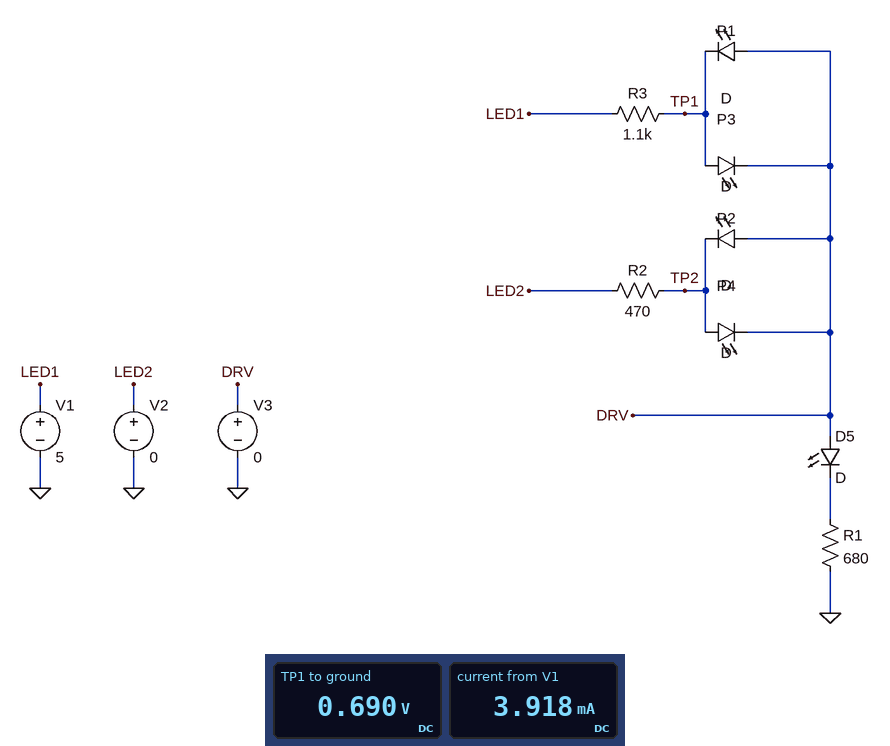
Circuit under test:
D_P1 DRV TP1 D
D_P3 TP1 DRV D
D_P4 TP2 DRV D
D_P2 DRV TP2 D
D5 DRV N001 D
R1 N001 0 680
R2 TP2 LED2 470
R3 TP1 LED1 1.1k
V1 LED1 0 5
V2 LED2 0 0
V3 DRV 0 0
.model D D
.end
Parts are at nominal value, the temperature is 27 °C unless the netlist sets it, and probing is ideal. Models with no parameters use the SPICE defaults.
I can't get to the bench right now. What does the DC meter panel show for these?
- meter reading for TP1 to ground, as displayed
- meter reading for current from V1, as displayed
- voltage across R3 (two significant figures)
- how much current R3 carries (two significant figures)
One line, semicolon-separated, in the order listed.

0.690 V; 3.918 mA; 4.3 V; 3.9 mA
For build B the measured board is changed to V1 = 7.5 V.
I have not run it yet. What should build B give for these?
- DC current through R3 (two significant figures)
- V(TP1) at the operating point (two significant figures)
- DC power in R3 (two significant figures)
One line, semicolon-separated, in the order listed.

6.2 mA; 700 mV; 42 mW
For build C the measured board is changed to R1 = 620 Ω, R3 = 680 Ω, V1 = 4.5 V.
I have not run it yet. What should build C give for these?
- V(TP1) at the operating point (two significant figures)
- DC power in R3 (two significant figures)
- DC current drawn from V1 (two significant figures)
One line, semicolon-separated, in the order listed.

700 mV; 21 mW; 5.6 mA
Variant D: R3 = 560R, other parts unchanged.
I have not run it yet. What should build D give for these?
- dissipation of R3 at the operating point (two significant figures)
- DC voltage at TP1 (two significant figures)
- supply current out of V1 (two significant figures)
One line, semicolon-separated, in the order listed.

33 mW; 710 mV; 7.7 mA
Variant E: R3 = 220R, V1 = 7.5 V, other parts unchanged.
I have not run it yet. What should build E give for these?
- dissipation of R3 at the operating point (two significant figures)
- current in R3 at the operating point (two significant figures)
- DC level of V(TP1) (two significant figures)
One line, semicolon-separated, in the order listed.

210 mW; 31 mA; 740 mV
